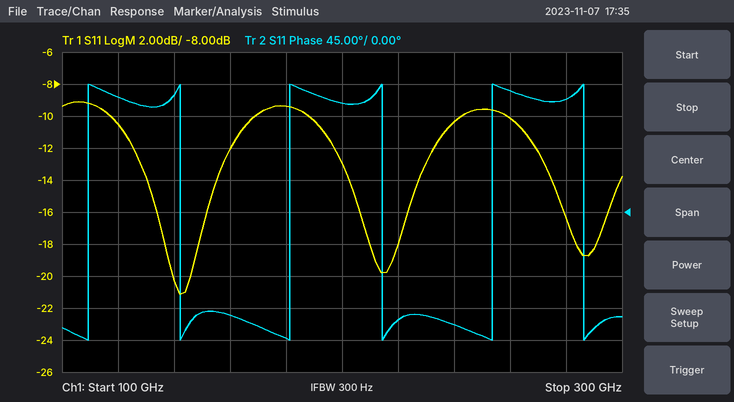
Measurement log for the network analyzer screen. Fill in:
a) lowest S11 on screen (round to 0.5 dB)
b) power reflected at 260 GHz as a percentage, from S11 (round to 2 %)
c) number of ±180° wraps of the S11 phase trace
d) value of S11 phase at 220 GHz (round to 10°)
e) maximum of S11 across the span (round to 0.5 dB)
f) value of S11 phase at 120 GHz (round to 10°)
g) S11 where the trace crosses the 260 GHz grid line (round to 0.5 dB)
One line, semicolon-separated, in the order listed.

-21.0 dB; 10 %; 6; -150°; -9.0 dB; 160°; -10.0 dB
